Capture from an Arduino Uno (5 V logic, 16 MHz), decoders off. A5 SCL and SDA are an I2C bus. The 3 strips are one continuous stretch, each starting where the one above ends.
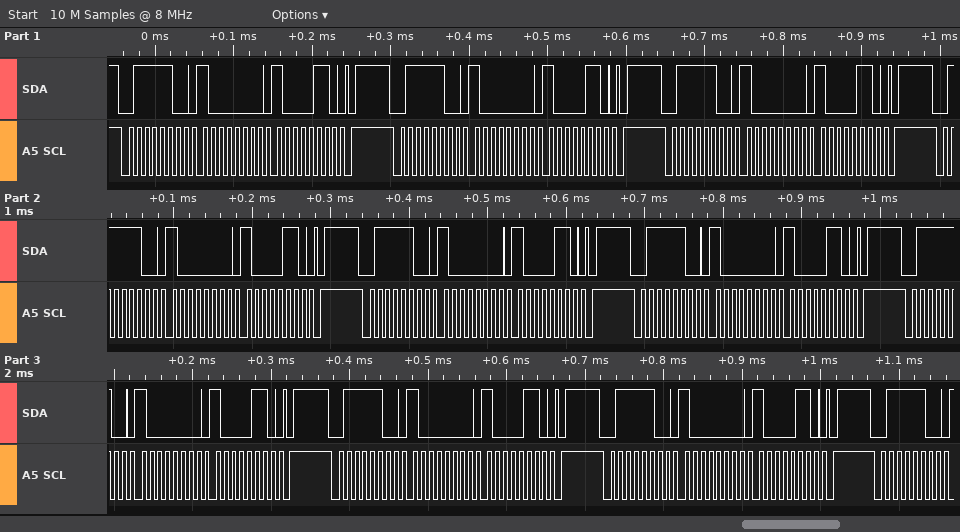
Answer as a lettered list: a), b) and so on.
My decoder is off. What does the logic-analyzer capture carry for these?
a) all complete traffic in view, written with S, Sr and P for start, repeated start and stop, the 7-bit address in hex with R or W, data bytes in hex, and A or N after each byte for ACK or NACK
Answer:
a) S 3EW A 80 A 86 A P S 3EW A 80 A 86 A P S 3EW A 80 A 86 A P S 3EW A 80 A 86 A P S 3EW A 80 A 86 A P S 3EW A 80 A 86 A P S 3EW A 80 A 86 A P S 3EW A 80 A 86 A P S 3EW A 80 A 86 A P S 3EW A
